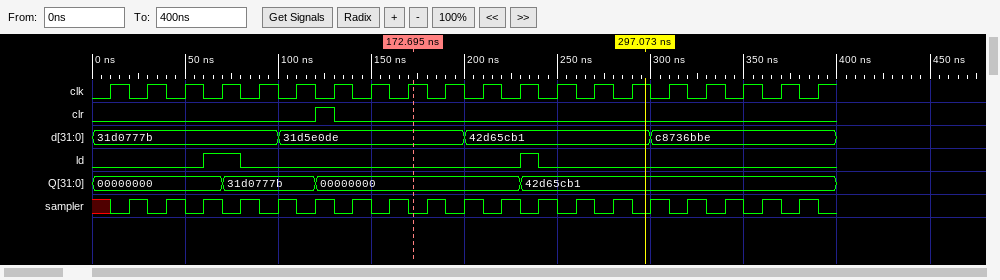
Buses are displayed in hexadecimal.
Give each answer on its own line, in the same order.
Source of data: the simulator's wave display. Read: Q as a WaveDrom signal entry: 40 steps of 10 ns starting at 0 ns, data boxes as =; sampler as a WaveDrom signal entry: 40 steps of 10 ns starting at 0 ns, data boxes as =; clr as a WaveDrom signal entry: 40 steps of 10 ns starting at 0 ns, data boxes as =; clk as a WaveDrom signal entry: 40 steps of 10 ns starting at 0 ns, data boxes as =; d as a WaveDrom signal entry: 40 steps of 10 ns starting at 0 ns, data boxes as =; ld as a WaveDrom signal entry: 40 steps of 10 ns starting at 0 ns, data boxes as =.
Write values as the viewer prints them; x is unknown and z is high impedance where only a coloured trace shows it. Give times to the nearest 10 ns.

{name: 'Q', wave: '=......=....=..........=................', data: '00000000 31d0777b 00000000 42d65cb1'}
{name: 'sampler', wave: 'x010101010101010101010101010101010101010'}
{name: 'clr', wave: '0...........10..........................'}
{name: 'clk', wave: '0101010101010101010101010101010101010101'}
{name: 'd', wave: '=.........=.........=.........=.........', data: '31d0777b 31d5e0de 42d65cb1 c8736bbe'}
{name: 'ld', wave: '0.....1.0..............10...............'}
